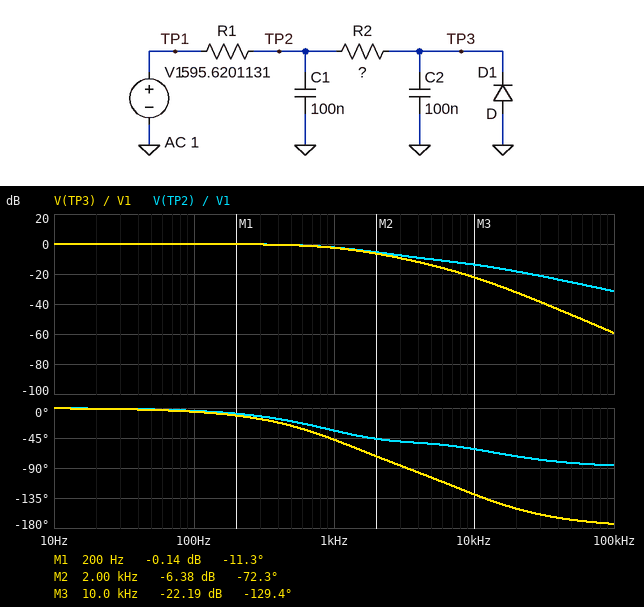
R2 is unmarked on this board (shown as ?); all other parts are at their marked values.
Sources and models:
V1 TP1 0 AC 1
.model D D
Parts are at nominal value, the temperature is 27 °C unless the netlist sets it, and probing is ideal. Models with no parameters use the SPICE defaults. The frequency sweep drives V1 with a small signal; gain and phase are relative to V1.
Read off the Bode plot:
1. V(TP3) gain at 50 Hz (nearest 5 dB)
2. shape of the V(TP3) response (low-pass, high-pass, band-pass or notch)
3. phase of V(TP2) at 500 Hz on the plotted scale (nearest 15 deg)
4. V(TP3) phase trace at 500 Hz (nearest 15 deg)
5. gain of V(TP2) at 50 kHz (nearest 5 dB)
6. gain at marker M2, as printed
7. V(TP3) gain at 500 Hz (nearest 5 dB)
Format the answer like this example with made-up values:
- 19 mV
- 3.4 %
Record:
- 0 dB
- low-pass
- -15 deg
- -30 deg
- -25 dB
- -6.38 dB
- 0 dB
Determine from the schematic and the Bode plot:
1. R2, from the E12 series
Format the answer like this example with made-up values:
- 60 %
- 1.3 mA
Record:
- 390 Ω
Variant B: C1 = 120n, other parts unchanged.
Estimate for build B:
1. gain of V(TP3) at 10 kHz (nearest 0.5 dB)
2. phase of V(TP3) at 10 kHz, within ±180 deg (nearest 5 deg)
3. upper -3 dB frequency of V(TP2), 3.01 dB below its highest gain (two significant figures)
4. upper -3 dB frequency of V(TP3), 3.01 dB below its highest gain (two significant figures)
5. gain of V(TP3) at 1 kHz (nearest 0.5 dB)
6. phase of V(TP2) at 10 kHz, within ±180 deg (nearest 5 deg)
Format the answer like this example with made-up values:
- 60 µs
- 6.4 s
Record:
- -23.5 dB
- -135 deg
- 1.1 kHz
- 1.0 kHz
- -3.0 dB
- -65 deg
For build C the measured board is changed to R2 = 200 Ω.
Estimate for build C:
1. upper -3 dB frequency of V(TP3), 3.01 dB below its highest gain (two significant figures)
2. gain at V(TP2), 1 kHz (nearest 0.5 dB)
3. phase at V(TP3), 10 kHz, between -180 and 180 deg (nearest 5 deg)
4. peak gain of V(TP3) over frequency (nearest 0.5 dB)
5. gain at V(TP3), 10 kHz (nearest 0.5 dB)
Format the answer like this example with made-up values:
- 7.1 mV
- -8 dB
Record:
- 1.2 kHz
- -2.0 dB
- -115 deg
- 0 dB
- -19.5 dB
